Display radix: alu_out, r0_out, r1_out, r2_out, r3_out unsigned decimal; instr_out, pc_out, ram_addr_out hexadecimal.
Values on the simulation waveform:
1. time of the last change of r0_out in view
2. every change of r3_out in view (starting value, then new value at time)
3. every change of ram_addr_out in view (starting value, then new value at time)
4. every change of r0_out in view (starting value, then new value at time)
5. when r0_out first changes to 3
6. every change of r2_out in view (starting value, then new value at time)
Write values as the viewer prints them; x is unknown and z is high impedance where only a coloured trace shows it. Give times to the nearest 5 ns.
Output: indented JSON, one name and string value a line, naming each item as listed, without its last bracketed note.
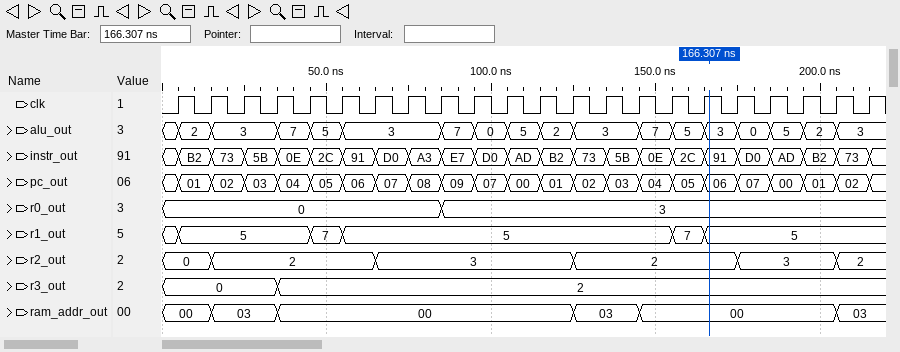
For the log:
{
  "time of the last change of r0_out in view": "85 ns",
  "every change of r3_out in view": "0, 2 at 35 ns",
  "every change of ram_addr_out in view": "00, 03 at 15 ns, 00 at 35 ns, 03 at 125 ns, 00 at 145 ns, 03 at 205 ns",
  "every change of r0_out in view": "0, 3 at 85 ns",
  "when r0_out first changes to 3": "85 ns",
  "every change of r2_out in view": "0, 2 at 15 ns, 3 at 65 ns, 2 at 125 ns, 3 at 175 ns, 2 at 205 ns"
}
